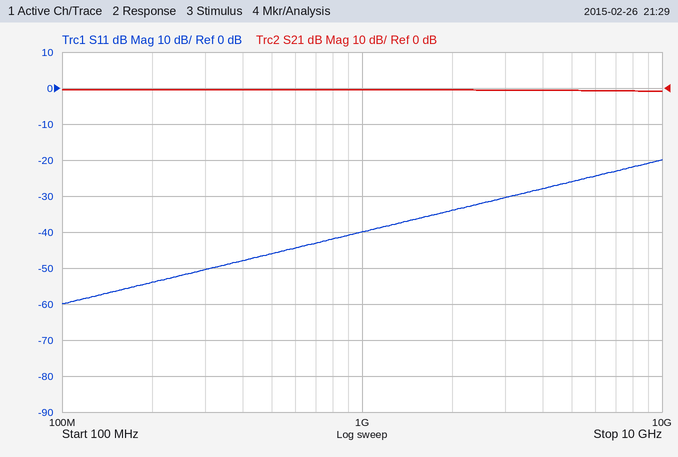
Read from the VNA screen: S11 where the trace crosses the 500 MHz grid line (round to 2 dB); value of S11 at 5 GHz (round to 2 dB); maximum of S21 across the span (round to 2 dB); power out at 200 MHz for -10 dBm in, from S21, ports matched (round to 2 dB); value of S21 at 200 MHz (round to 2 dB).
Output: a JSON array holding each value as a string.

["-46 dB", "-26 dB", "0 dB", "-10 dBm", "0 dB"]
